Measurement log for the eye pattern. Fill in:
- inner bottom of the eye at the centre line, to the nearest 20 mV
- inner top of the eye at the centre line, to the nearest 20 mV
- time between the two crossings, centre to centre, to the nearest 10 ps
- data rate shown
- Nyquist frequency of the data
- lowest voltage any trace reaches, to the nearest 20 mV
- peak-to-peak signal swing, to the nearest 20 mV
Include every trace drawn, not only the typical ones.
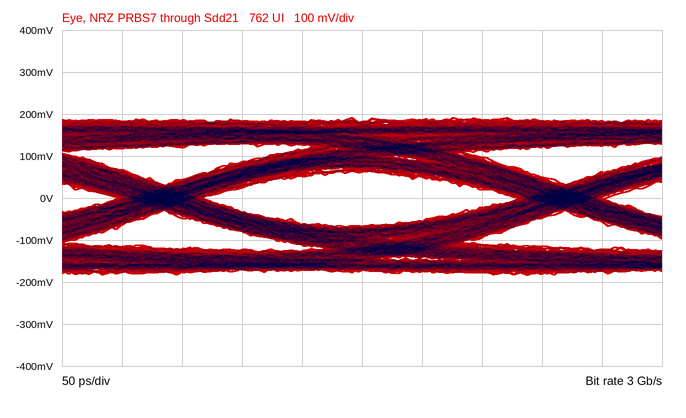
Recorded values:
-60 mV
60 mV
330 ps
3 Gb/s
1.5 GHz
-180 mV
380 mV
